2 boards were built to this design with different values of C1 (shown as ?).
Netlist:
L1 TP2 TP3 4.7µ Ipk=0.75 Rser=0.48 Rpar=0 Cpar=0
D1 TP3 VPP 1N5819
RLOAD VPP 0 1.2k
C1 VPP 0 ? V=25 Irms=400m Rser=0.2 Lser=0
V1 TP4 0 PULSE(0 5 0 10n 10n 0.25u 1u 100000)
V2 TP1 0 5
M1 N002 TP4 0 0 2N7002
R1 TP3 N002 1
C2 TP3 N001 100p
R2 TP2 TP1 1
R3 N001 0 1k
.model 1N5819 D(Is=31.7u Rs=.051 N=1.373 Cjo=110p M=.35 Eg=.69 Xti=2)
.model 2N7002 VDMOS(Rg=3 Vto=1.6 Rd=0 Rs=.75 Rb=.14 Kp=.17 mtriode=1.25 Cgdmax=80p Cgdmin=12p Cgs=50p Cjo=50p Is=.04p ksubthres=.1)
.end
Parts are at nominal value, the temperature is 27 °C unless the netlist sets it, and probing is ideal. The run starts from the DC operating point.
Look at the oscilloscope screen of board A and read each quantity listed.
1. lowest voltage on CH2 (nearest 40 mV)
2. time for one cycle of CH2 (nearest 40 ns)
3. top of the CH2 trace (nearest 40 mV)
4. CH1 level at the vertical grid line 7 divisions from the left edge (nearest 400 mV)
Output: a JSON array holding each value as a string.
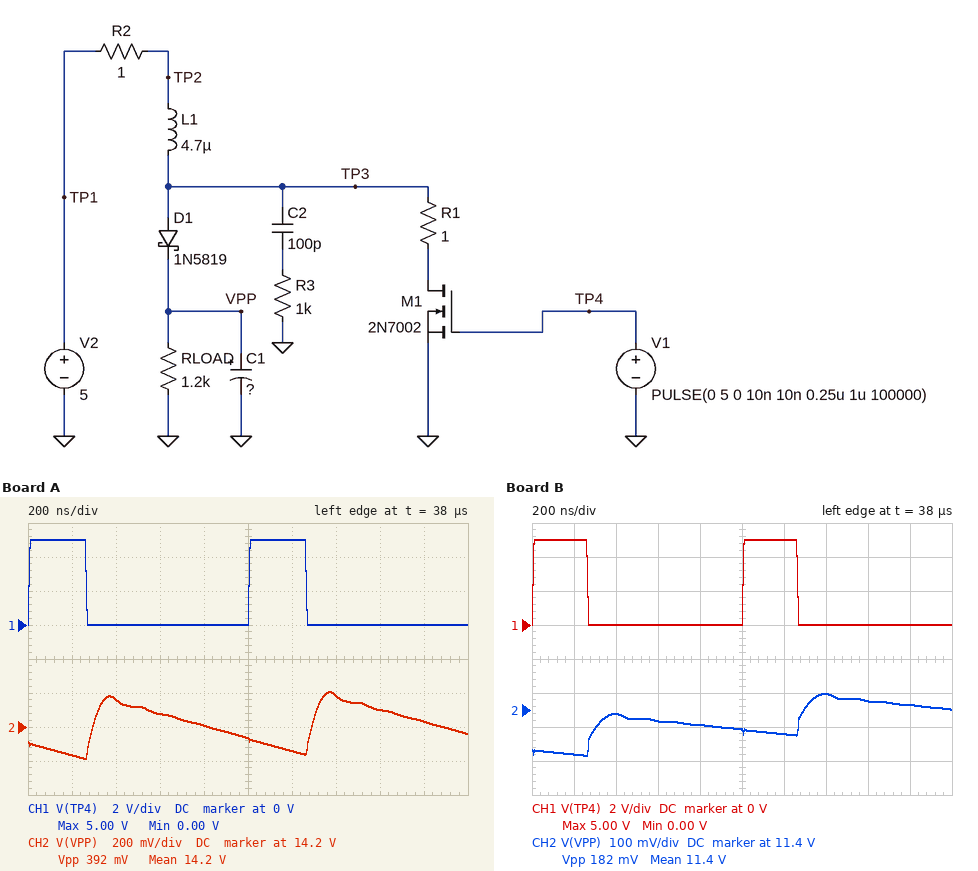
["14.00 V", "1.00 µs", "14.40 V", "0 V"]
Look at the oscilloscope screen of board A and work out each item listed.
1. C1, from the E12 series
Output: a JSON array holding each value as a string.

["33 nF"]
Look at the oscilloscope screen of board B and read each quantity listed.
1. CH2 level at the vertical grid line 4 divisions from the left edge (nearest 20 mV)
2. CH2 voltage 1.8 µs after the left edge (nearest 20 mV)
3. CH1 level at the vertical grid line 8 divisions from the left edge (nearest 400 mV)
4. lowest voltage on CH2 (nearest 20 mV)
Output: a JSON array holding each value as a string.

["11.36 V", "11.42 V", "0 V", "11.26 V"]
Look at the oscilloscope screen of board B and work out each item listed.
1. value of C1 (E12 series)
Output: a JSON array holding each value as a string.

["150 nF"]
